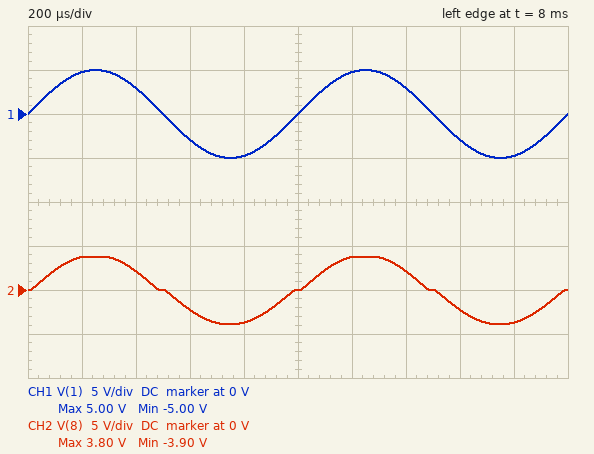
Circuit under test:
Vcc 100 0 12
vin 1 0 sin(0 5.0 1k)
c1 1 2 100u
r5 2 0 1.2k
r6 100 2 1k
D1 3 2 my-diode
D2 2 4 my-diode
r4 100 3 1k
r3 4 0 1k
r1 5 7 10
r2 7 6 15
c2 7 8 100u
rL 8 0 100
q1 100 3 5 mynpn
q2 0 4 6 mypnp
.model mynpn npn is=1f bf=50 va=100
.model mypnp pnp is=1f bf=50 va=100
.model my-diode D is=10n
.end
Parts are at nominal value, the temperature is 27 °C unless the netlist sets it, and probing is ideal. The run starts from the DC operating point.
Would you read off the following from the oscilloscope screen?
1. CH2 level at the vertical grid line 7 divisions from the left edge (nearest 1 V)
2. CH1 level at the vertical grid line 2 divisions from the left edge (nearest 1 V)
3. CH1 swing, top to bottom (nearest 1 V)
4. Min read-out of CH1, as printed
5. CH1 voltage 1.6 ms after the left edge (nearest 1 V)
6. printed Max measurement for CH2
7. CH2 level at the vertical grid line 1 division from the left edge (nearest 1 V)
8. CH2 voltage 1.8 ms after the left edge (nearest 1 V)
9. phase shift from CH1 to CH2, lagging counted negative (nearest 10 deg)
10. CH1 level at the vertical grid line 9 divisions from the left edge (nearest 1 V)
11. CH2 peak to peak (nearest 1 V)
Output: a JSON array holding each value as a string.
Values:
["2 V", "3 V", "10 V", "-5.00 V", "-3 V", "3.80 V", "4 V", "-4 V", "0 deg", "-5 V", "8 V"]
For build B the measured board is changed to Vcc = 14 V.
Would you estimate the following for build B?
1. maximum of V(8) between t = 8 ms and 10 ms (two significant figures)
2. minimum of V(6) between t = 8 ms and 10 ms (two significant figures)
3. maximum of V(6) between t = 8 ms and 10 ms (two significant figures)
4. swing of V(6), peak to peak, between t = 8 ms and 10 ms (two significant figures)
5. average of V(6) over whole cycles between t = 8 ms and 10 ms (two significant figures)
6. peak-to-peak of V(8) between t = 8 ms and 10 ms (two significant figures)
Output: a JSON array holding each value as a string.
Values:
["4.0 V", "2.8 V", "11 V", "8.6 V", "7.2 V", "8.0 V"]
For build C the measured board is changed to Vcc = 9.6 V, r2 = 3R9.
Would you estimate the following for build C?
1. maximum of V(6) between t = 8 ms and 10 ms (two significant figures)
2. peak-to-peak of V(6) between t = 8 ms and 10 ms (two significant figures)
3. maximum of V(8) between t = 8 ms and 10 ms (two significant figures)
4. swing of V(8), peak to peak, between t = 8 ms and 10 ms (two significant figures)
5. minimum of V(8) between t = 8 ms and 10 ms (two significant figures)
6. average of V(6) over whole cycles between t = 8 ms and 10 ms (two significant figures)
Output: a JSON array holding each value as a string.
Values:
["7.9 V", "6.5 V", "3.0 V", "6.4 V", "-3.4 V", "4.8 V"]
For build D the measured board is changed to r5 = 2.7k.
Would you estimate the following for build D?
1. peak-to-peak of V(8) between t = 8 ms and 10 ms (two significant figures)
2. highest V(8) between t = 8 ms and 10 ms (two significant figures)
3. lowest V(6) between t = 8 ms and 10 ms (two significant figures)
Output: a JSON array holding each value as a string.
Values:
["7.1 V", "3.2 V", "2.6 V"]
